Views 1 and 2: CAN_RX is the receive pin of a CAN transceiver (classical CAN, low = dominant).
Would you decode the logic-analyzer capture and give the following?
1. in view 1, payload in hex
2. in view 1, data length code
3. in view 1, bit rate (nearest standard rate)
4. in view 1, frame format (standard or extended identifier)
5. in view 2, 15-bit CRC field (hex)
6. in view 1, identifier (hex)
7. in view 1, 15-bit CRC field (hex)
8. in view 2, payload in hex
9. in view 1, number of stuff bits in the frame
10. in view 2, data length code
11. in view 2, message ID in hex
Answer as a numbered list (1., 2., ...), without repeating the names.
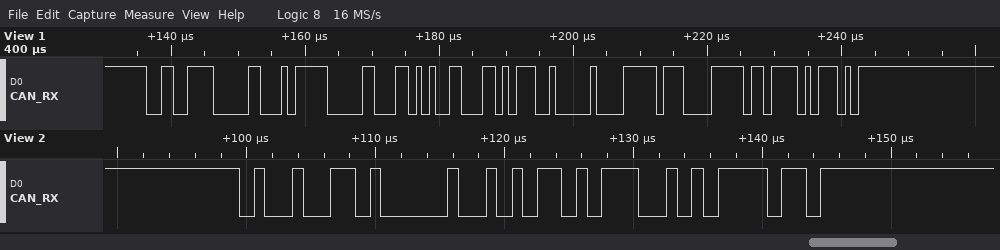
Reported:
1. BE 11 A9 8D 72 00 FF 0F
2. 8
3. 1000 kbit/s
4. standard
5. 0x72BD
6. 0x33C
7. 0x77AE
8. 5A
9. 6
10. 1
11. 0x49A
